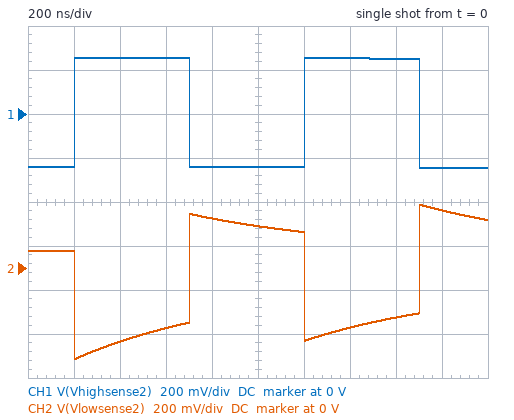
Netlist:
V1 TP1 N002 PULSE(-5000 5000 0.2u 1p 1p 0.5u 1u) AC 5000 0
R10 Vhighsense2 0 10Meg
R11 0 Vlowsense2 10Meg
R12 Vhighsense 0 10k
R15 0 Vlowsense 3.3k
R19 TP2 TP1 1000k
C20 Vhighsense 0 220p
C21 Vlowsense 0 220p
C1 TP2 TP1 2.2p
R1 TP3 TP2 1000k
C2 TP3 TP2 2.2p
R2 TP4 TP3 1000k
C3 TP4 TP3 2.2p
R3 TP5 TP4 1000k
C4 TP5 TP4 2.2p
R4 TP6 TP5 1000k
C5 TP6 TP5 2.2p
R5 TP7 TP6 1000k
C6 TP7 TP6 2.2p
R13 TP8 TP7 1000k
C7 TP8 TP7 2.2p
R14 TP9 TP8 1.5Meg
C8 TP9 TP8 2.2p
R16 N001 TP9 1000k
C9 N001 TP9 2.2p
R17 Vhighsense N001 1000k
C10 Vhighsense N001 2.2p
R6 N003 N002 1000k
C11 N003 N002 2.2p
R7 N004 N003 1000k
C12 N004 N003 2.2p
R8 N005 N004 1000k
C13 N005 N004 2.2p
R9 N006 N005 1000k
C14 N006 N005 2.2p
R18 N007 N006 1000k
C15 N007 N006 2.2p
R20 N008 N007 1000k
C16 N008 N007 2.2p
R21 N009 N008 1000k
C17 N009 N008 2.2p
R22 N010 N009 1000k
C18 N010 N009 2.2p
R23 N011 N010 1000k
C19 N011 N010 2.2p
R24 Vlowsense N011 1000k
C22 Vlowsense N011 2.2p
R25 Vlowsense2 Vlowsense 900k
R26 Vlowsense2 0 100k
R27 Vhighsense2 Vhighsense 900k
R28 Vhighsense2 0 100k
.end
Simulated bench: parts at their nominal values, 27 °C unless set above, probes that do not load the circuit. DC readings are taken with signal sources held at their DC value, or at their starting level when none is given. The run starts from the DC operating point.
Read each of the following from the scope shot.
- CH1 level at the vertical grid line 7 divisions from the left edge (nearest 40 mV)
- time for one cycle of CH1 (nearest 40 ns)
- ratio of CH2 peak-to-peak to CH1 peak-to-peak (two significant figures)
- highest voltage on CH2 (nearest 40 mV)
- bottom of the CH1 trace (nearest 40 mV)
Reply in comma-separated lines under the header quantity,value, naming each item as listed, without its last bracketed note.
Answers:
quantity,value
CH1 level at the vertical grid line 7 divisions from the left edge,240 mV
time for one cycle of CH1,1.00 µs
ratio of CH2 peak-to-peak to CH1 peak-to-peak,1.4
highest voltage on CH2,280 mV
bottom of the CH1 trace,-240 mV
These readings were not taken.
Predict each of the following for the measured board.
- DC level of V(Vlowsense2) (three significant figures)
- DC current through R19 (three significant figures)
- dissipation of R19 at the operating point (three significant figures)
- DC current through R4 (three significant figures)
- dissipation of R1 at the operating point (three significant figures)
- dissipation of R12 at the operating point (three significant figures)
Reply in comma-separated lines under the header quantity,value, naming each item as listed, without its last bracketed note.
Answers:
quantity,value
DC level of V(Vlowsense2),79.5 mV
DC current through R19,244 µA
dissipation of R19 at the operating point,59.4 mW
DC current through R4,244 µA
dissipation of R1 at the operating point,59.4 mW
dissipation of R12 at the operating point,582 µW
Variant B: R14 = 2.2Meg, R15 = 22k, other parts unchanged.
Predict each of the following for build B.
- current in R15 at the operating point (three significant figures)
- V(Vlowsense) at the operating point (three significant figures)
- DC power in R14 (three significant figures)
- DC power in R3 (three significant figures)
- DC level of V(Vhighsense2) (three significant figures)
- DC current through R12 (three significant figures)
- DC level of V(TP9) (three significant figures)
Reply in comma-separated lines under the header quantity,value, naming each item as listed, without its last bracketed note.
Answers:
quantity,value
current in R15 at the operating point,230 µA
V(Vlowsense) at the operating point,5.07 V
DC power in R14,122 mW
DC power in R3,55.5 mW
DC level of V(Vhighsense2),-231 mV
DC current through R12,233 µA
DC level of V(TP9),-473 V
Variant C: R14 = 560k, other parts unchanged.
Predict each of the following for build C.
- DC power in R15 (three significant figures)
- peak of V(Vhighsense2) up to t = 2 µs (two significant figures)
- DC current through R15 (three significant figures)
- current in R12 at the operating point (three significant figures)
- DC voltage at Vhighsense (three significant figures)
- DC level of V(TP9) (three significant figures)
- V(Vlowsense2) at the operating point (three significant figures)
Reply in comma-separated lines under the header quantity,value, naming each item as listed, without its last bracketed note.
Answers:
quantity,value
DC power in R15,214 µW
peak of V(Vhighsense2) up to t = 2 µs,250 mV
DC current through R15,255 µA
current in R12 at the operating point,253 µA
DC voltage at Vhighsense,-2.53 V
DC level of V(TP9),-513 V
V(Vlowsense2) at the operating point,83.3 mV
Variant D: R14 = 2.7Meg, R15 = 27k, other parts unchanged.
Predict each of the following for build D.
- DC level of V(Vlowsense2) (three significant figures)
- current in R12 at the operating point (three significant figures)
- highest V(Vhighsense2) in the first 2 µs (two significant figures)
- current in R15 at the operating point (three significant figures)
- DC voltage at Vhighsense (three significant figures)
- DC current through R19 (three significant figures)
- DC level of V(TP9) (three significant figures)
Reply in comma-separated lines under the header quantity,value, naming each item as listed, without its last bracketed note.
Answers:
quantity,value
DC level of V(Vlowsense2),599 mV
current in R12 at the operating point,228 µA
highest V(Vhighsense2) in the first 2 µs,270 mV
current in R15 at the operating point,224 µA
DC voltage at Vhighsense,-2.28 V
DC current through R19,230 µA
DC level of V(TP9),-462 V
